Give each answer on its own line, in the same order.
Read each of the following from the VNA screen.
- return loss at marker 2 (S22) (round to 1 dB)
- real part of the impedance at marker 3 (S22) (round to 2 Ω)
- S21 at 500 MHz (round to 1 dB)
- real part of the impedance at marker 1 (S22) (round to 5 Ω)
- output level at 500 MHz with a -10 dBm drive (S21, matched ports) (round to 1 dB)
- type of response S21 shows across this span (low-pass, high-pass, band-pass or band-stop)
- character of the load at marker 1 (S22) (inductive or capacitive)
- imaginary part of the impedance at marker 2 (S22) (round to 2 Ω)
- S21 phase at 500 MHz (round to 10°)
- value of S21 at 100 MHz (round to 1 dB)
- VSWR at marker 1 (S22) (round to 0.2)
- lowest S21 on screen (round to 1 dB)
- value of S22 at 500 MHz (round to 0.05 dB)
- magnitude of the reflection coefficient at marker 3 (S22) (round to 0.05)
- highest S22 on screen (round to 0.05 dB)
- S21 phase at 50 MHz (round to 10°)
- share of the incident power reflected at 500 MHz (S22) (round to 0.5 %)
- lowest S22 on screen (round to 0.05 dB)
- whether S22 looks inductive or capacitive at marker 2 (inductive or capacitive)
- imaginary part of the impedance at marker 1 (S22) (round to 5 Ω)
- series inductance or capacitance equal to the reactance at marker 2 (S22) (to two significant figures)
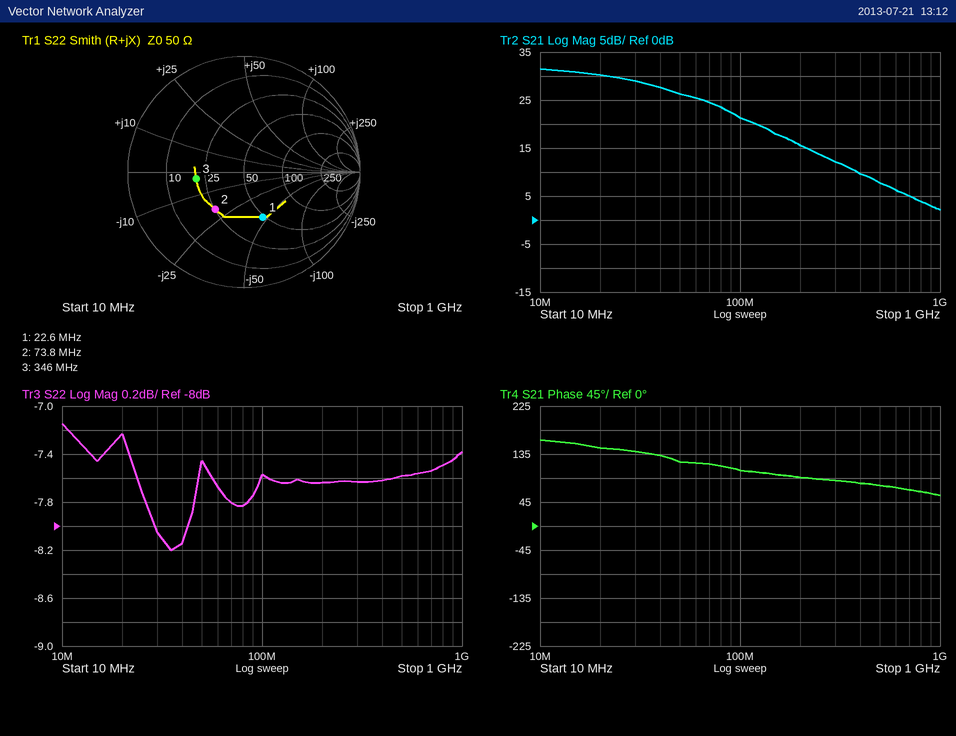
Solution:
8 dB
20 Ω
8 dB
50 Ω
-2 dBm
low-pass
capacitive
-20 Ω
80°
21 dB
2.4
2 dB
-7.60 dB
0.40
-7.15 dB
120°
17.5 %
-8.20 dB
capacitive
-45 Ω
110 pF
